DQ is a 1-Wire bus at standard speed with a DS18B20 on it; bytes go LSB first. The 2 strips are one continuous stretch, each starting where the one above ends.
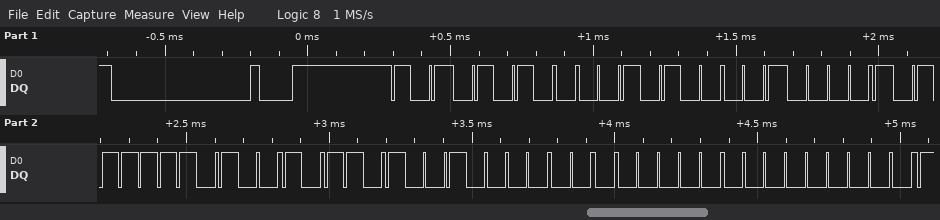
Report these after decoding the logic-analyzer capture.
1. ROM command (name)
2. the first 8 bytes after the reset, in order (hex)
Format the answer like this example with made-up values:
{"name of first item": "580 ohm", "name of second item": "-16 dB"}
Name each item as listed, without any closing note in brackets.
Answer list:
{"ROM command": "Match ROM", "the first 8 bytes after the reset, in order": "55 28 84 7E 69 09 00 00"}
